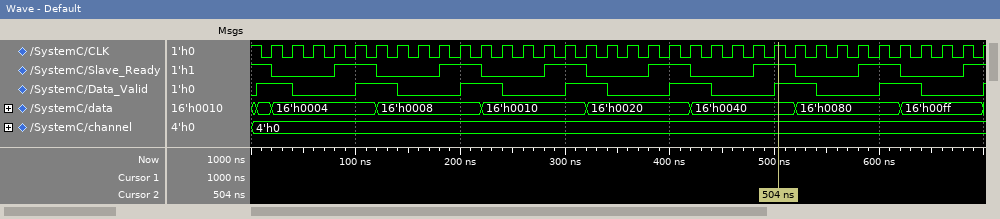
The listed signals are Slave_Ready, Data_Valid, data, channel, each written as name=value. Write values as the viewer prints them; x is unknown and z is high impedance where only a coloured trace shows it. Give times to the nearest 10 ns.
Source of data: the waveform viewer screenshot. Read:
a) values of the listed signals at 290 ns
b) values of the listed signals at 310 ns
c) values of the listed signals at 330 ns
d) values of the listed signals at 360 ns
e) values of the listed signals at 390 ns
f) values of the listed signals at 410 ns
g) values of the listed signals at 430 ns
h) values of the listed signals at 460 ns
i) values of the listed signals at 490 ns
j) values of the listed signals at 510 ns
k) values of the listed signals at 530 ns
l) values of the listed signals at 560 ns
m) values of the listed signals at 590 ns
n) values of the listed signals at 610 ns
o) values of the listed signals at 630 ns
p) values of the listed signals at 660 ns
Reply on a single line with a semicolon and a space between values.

Slave_Ready=1, Data_Valid=0, data=16'h0010, channel=4'h0; Slave_Ready=1, Data_Valid=1, data=16'h0010, channel=4'h0; Slave_Ready=0, Data_Valid=1, data=16'h0020, channel=4'h0; Slave_Ready=0, Data_Valid=0, data=16'h0020, channel=4'h0; Slave_Ready=1, Data_Valid=0, data=16'h0020, channel=4'h0; Slave_Ready=1, Data_Valid=1, data=16'h0020, channel=4'h0; Slave_Ready=0, Data_Valid=1, data=16'h0040, channel=4'h0; Slave_Ready=0, Data_Valid=0, data=16'h0040, channel=4'h0; Slave_Ready=1, Data_Valid=0, data=16'h0040, channel=4'h0; Slave_Ready=1, Data_Valid=1, data=16'h0040, channel=4'h0; Slave_Ready=0, Data_Valid=1, data=16'h0080, channel=4'h0; Slave_Ready=0, Data_Valid=0, data=16'h0080, channel=4'h0; Slave_Ready=1, Data_Valid=0, data=16'h0080, channel=4'h0; Slave_Ready=1, Data_Valid=1, data=16'h0080, channel=4'h0; Slave_Ready=0, Data_Valid=1, data=16'h00ff, channel=4'h0; Slave_Ready=0, Data_Valid=0, data=16'h00ff, channel=4'h0
